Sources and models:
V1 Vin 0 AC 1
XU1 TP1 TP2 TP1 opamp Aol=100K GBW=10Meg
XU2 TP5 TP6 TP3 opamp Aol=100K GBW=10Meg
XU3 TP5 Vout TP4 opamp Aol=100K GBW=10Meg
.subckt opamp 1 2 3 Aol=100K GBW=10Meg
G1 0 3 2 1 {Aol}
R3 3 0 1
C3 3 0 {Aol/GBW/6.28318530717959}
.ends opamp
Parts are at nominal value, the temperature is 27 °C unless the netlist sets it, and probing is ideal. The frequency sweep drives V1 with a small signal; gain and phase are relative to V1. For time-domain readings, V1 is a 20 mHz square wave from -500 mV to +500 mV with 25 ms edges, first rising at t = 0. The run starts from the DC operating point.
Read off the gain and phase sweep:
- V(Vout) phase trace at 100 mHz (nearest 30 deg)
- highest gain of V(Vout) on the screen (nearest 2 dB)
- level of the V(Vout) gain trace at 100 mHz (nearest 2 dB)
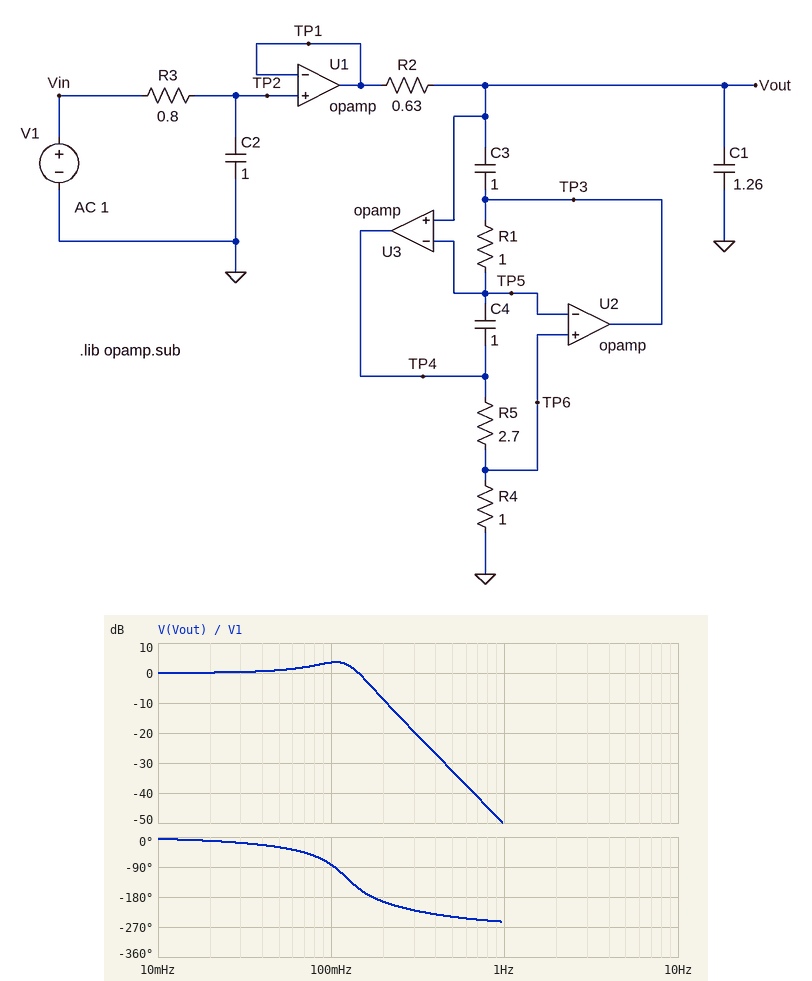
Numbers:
-90 deg
4 dB
4 dB
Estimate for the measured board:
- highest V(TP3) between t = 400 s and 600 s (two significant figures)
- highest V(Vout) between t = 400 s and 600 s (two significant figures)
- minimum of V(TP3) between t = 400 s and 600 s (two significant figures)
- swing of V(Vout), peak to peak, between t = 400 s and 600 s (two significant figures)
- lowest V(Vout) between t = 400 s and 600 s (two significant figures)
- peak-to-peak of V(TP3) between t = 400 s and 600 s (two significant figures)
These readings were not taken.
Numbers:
1.2 V
800 mV
-1.2 V
1.6 V
-800 mV
2.4 V
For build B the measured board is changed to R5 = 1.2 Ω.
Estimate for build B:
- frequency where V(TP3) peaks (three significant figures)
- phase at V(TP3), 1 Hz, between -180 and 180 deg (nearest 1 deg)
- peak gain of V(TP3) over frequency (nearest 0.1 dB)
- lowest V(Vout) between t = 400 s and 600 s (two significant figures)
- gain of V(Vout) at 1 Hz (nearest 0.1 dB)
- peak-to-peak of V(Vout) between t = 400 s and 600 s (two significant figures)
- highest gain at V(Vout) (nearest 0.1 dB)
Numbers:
151 mHz
29 deg
3.4 dB
-620 mV
-43.5 dB
1.2 V
0.3 dB
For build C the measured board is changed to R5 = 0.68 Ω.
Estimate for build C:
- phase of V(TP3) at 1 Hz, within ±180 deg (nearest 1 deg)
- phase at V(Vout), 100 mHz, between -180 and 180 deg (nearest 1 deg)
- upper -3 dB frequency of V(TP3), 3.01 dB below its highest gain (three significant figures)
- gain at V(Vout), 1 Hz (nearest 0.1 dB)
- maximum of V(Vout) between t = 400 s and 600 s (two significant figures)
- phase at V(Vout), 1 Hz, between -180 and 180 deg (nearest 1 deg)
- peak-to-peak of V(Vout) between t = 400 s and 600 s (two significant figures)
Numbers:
42 deg
-58 deg
256 mHz
-38.6 dB
520 mV
119 deg
1.0 V
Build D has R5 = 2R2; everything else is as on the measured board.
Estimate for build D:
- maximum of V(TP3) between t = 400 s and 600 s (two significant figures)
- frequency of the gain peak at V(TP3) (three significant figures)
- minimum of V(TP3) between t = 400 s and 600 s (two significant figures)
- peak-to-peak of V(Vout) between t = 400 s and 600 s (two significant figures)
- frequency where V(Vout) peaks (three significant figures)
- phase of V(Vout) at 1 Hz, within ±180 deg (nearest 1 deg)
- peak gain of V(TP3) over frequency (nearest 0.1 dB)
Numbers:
1.1 V
127 mHz
-1.1 V
1.5 V
113 mHz
107 deg
8.4 dB
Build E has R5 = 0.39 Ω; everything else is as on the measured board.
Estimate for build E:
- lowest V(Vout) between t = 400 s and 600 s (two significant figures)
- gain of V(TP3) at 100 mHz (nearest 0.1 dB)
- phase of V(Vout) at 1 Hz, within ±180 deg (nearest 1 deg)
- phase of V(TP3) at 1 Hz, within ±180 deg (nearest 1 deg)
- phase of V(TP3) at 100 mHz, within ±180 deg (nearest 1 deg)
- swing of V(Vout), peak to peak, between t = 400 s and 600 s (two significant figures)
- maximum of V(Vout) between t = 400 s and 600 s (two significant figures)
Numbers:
-500 mV
-1.0 dB
131 deg
63 deg
-69 deg
1.0 V
500 mV
